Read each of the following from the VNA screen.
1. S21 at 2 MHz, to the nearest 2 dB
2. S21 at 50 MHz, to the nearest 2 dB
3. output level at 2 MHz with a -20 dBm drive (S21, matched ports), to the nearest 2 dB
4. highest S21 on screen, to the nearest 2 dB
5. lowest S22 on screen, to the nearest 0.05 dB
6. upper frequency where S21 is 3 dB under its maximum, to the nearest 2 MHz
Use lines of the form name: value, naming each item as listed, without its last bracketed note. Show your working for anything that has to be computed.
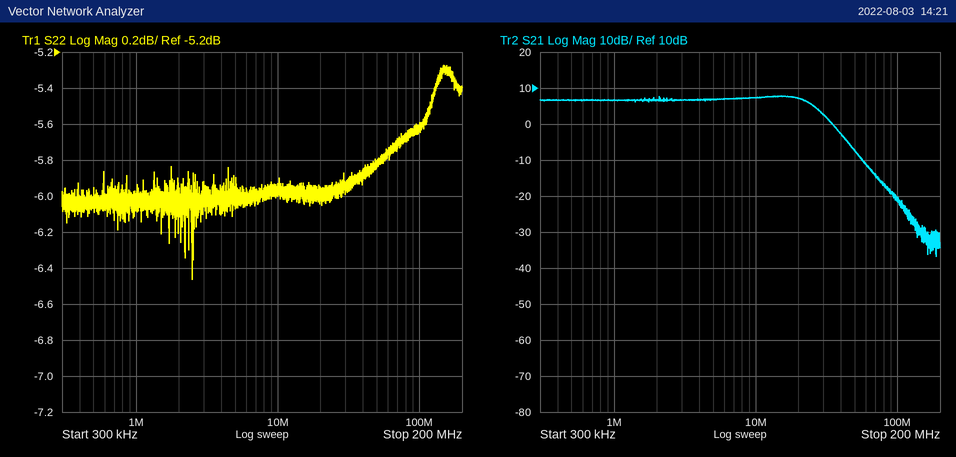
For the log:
S21 at 2 MHz, to the nearest 2 dB: 6 dB
S21 at 50 MHz, to the nearest 2 dB: -8 dB
output level at 2 MHz with a -20 dBm drive (S21, matched ports), to the nearest 2 dB: -20 dBm + (6 dB) = -14 dBm
highest S21 on screen, to the nearest 2 dB: 8 dB
lowest S22 on screen, to the nearest 0.05 dB: -6.45 dB
upper frequency where S21 is 3 dB under its maximum, to the nearest 2 MHz: 26 MHz
